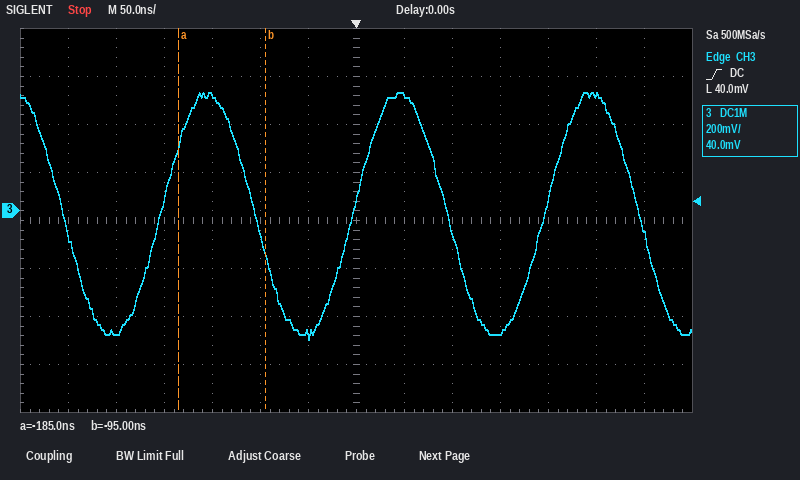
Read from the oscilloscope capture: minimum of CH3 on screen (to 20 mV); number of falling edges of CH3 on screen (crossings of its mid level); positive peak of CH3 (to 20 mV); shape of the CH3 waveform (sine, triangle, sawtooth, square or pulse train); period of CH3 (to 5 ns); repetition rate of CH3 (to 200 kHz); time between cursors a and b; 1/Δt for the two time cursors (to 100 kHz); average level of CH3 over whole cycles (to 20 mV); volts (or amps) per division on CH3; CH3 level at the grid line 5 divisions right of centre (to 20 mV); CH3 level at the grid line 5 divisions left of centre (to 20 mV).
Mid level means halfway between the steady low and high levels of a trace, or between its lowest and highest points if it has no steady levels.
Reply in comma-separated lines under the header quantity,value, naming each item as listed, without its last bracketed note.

quantity,value
minimum of CH3 on screen,-540 mV
number of falling edges of CH3 on screen,4
positive peak of CH3,500 mV
shape of the CH3 waveform,sine
period of CH3,200 ns
repetition rate of CH3,5.0 MHz
time between cursors a and b,90 ns
1/Δt for the two time cursors,11.1 MHz
average level of CH3 over whole cycles,-20 mV
volts (or amps) per division on CH3,200 mV
CH3 level at the grid line 5 divisions right of centre,480 mV
CH3 level at the grid line 5 divisions left of centre,-520 mV
